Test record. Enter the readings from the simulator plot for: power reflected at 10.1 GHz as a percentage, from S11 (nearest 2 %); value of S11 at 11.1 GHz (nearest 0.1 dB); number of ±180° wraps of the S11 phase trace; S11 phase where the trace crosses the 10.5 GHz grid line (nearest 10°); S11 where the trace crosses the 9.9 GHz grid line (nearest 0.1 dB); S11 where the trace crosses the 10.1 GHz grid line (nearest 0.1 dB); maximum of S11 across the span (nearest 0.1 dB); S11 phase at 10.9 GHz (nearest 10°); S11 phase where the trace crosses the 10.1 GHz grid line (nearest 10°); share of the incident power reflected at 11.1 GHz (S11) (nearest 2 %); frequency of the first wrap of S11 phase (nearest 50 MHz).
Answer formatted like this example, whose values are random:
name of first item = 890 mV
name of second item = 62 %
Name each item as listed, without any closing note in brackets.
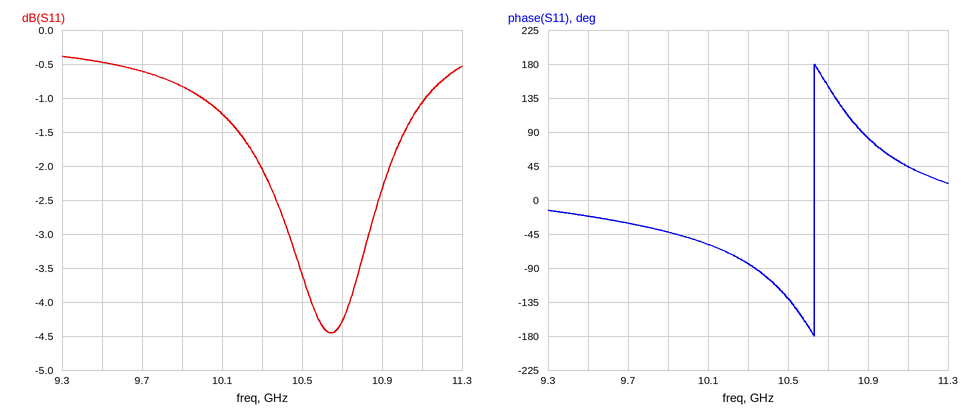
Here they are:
power reflected at 10.1 GHz as a percentage, from S11 = 76 %
value of S11 at 11.1 GHz = -1.1 dB
number of ±180° wraps of the S11 phase trace = 1
S11 phase where the trace crosses the 10.5 GHz grid line = -130°
S11 where the trace crosses the 9.9 GHz grid line = -0.8 dB
S11 where the trace crosses the 10.1 GHz grid line = -1.2 dB
maximum of S11 across the span = -0.4 dB
S11 phase at 10.9 GHz = 80°
S11 phase where the trace crosses the 10.1 GHz grid line = -60°
share of the incident power reflected at 11.1 GHz (S11) = 78 %
frequency of the first wrap of S11 phase = 10.65 GHz
